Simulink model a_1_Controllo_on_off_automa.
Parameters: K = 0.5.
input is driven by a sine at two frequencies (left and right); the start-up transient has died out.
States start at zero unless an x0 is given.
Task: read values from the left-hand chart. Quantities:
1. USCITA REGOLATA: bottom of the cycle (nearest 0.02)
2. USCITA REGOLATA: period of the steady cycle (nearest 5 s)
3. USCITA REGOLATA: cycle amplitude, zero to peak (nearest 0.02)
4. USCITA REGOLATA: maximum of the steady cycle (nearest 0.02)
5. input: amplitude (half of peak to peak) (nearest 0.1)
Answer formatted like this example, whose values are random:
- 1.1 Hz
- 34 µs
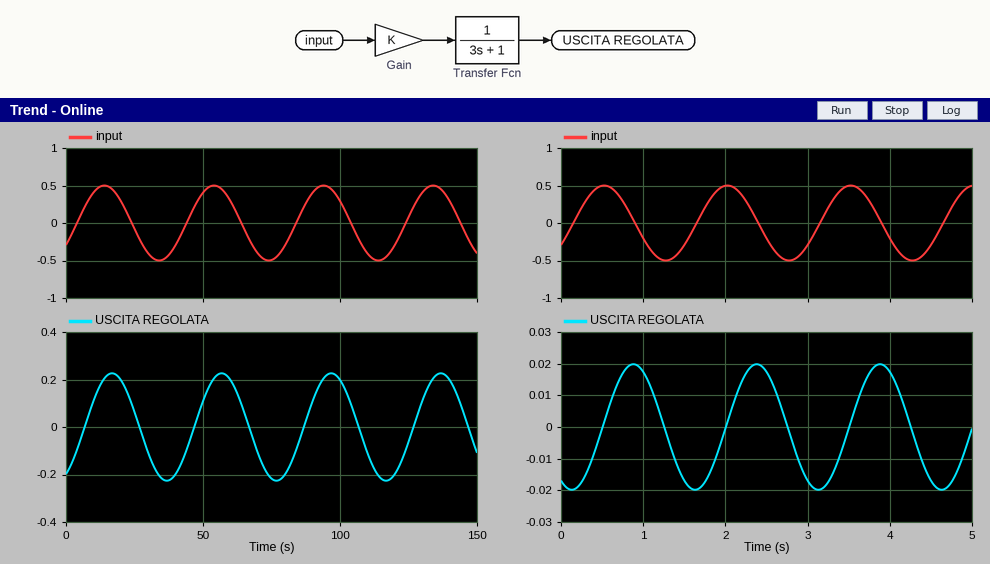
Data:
- -0.22
- 40 s
- 0.22
- 0.22
- 0.5
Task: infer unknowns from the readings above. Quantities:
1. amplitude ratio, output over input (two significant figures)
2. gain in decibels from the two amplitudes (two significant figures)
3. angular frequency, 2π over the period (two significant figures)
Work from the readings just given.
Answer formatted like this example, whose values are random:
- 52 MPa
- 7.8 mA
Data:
- 0.44
- -7.1 dB
- 0.16 rad/s
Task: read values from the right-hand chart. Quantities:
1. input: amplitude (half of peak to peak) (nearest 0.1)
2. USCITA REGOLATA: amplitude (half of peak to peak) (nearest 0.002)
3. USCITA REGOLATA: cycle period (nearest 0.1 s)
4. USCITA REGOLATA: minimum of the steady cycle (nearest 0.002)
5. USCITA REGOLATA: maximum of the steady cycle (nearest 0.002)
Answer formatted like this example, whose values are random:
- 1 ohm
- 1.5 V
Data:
- 0.5
- 0.020
- 1.5 s
- -0.020
- 0.020
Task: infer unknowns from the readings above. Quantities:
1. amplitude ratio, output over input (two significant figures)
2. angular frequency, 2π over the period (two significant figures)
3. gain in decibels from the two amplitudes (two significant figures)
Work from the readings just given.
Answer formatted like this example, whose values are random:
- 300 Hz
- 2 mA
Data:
- 0.040
- 4.2 rad/s
- -28 dB
